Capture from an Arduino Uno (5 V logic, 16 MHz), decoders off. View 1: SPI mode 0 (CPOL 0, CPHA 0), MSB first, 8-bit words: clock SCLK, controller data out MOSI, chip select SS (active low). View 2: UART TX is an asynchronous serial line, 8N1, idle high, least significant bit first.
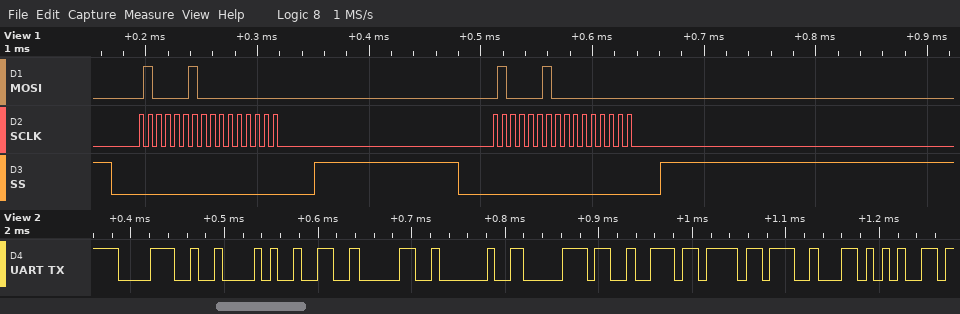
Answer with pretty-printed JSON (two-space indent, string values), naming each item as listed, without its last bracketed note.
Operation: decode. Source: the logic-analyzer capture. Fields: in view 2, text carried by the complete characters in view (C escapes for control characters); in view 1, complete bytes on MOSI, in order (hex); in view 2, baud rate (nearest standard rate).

{
  "in view 2, text carried by the complete characters in view": "\"8B20 probe\"",
  "in view 1, complete bytes on MOSI, in order": "42 00 42 00",
  "in view 2, baud rate": "115200 baud"
}
